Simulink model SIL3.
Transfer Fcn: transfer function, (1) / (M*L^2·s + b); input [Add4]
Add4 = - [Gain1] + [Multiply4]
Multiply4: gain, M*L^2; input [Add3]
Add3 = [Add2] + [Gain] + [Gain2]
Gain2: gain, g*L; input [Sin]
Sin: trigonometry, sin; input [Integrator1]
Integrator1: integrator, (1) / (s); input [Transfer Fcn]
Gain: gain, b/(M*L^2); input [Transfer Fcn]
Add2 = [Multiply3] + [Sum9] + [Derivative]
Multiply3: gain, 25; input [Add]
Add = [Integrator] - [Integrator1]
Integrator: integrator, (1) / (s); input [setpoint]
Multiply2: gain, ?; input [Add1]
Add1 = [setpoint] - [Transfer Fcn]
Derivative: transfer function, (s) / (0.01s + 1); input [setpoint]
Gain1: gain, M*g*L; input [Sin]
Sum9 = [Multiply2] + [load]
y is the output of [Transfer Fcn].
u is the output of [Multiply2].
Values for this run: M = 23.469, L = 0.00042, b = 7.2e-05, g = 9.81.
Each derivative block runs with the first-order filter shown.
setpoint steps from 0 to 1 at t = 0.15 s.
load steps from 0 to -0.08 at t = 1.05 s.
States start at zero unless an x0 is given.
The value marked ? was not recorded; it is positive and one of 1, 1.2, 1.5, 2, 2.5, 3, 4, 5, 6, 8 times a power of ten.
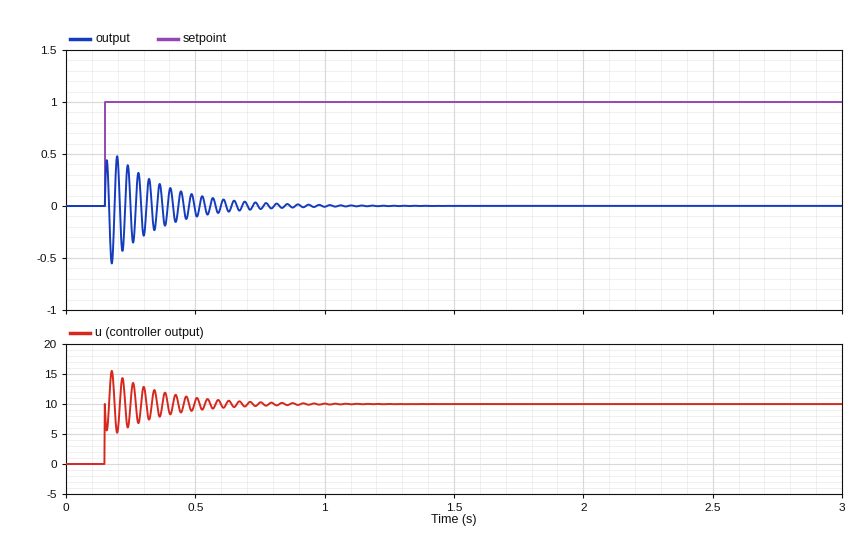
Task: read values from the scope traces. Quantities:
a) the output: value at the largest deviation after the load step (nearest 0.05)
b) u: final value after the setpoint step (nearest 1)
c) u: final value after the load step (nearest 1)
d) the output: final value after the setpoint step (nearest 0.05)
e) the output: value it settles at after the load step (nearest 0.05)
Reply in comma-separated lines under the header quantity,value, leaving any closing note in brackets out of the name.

quantity,value
the output: value at the largest deviation after the load step,0.00
u: final value after the setpoint step,10
u: final value after the load step,10
the output: final value after the setpoint step,0.00
the output: value it settles at after the load step,0.00
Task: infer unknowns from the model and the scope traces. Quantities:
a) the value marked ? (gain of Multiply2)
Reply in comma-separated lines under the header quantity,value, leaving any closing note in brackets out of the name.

quantity,value
the value marked ?,10
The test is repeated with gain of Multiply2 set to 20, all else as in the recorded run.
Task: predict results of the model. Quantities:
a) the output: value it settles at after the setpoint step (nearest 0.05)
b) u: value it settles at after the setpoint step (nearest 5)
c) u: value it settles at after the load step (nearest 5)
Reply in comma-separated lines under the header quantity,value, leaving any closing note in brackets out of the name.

quantity,value
the output: value it settles at after the setpoint step,0.00
u: value it settles at after the setpoint step,20
u: value it settles at after the load step,20
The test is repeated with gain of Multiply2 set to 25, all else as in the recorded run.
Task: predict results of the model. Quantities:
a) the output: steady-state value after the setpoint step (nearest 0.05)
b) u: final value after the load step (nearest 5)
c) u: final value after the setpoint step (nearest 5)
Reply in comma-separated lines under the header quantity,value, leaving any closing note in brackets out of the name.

quantity,value
the output: steady-state value after the setpoint step,0.00
u: final value after the load step,25
u: final value after the setpoint step,25
